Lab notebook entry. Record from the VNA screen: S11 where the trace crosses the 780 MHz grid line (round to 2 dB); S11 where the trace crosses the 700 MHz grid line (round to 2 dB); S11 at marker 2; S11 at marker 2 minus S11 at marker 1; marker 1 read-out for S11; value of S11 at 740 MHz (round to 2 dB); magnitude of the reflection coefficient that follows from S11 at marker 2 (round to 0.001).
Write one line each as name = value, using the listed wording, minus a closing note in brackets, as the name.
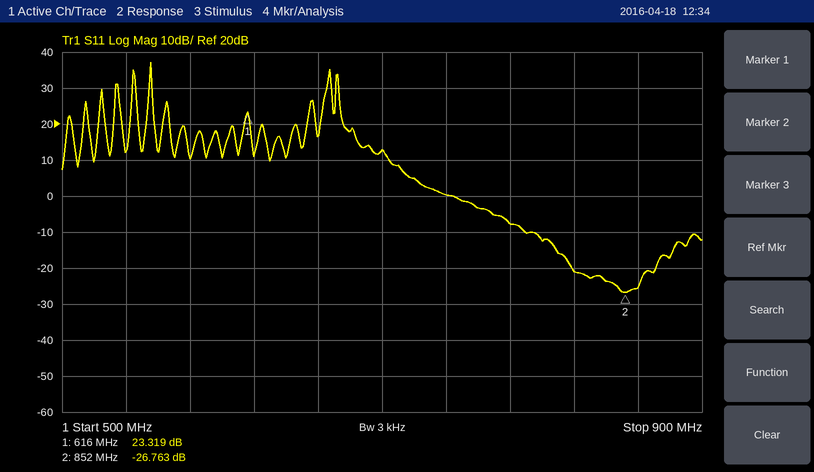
S11 where the trace crosses the 780 MHz grid line = -8 dB
S11 where the trace crosses the 700 MHz grid line = 12 dB
S11 at marker 2 = -26.763 dB
S11 at marker 2 minus S11 at marker 1 = -50.082 dB
marker 1 read-out for S11 = 23.319 dB
value of S11 at 740 MHz = 0 dB
magnitude of the reflection coefficient that follows from S11 at marker 2 = 0.046
